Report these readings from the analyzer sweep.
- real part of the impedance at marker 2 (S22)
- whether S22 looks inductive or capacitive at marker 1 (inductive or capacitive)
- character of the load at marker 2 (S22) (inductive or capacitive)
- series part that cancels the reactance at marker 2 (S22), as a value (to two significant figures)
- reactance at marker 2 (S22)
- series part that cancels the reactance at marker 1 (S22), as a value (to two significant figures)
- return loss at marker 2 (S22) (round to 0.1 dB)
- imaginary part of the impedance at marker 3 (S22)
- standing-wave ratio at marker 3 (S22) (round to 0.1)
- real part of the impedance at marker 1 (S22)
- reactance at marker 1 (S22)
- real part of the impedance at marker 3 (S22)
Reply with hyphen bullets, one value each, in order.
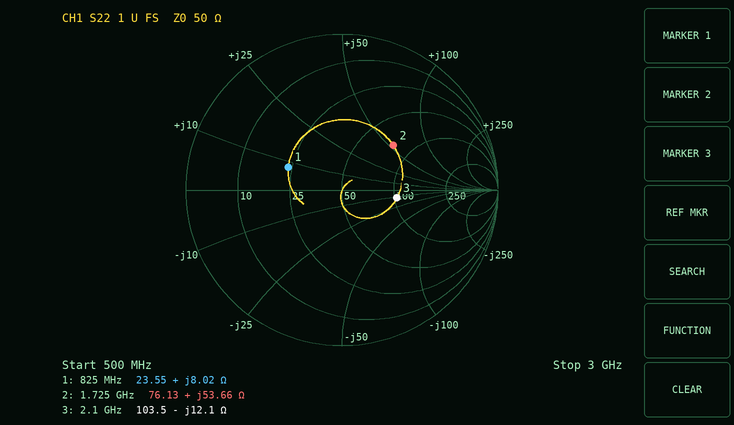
- 76.13 Ω
- inductive
- inductive
- 1.7 pF
- +53.66 Ω
- 24 pF
- 7.2 dB
- -12.1 Ω
- 2.1
- 23.55 Ω
- +8.02 Ω
- 103.5 Ω
